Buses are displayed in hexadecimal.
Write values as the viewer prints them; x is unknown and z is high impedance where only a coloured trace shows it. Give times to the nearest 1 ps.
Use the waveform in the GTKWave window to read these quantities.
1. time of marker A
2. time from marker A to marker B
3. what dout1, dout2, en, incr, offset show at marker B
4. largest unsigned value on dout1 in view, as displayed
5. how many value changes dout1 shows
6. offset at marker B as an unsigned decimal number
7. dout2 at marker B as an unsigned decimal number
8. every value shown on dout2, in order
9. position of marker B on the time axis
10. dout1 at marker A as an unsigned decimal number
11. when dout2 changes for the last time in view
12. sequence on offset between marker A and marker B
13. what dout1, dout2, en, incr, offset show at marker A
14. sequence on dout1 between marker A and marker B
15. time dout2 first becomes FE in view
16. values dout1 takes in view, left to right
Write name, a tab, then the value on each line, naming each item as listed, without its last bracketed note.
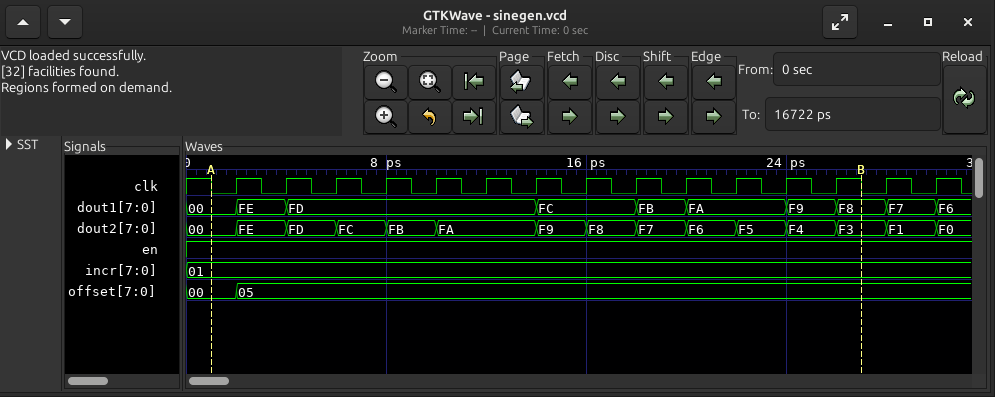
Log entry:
time of marker A	1 ps
time from marker A to marker B	26 ps
what dout1, dout2, en, incr, offset show at marker B	dout1=F8, dout2=F3, en=1, incr=01, offset=05
largest unsigned value on dout1 in view, as displayed	FE
how many value changes dout1 shows	9
offset at marker B as an unsigned decimal number	5
dout2 at marker B as an unsigned decimal number	243
every value shown on dout2, in order	00, FE, FD, FC, FB, FA, F9, F8, F7, F6, F5, F4, F3, F1, F0
position of marker B on the time axis	27 ps
dout1 at marker A as an unsigned decimal number	0
when dout2 changes for the last time in view	30 ps
sequence on offset between marker A and marker B	00, 05
what dout1, dout2, en, incr, offset show at marker A	dout1=00, dout2=00, en=1, incr=01, offset=00
sequence on dout1 between marker A and marker B	00, FE, FD, FC, FB, FA, F9, F8
time dout2 first becomes FE in view	2 ps
values dout1 takes in view, left to right	00, FE, FD, FC, FB, FA, F9, F8, F7, F6
